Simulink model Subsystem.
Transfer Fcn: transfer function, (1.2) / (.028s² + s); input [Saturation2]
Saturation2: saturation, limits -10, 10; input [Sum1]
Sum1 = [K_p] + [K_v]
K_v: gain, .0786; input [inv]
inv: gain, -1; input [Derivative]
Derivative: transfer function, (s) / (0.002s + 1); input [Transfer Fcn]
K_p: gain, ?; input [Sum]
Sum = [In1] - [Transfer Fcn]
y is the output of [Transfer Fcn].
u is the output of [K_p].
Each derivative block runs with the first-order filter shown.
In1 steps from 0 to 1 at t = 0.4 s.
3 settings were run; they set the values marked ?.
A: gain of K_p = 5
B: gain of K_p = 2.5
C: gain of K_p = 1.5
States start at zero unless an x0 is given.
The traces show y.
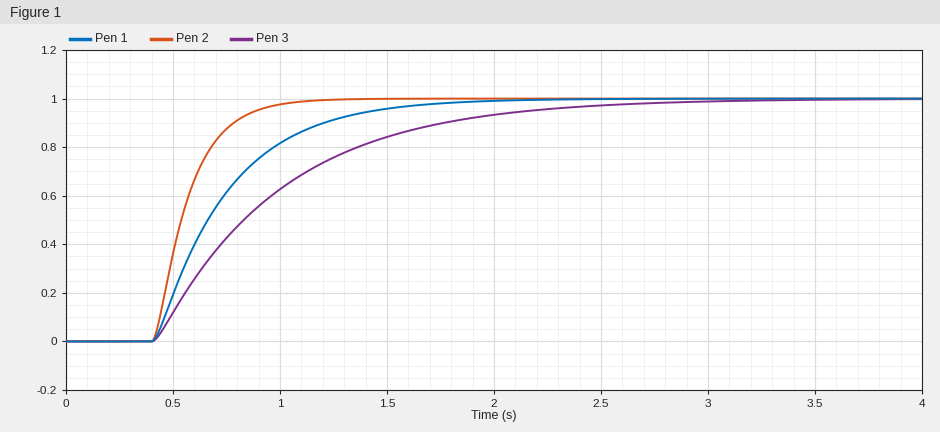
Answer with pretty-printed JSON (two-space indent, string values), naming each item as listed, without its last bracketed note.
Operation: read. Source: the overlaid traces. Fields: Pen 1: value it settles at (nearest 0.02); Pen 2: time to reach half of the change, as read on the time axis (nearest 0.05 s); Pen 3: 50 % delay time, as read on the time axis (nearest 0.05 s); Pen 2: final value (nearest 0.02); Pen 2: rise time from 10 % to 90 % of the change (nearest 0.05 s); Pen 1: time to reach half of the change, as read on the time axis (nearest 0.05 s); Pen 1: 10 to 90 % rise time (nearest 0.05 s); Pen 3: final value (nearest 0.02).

{
  "Pen 1: value it settles at": "1.00",
  "Pen 2: time to reach half of the change, as read on the time axis": "0.55 s",
  "Pen 3: 50 % delay time, as read on the time axis": "0.85 s",
  "Pen 2: final value": "1.00",
  "Pen 2: rise time from 10 % to 90 % of the change": "0.35 s",
  "Pen 1: time to reach half of the change, as read on the time axis": "0.65 s",
  "Pen 1: 10 to 90 % rise time": "0.75 s",
  "Pen 3: final value": "1.00"
}
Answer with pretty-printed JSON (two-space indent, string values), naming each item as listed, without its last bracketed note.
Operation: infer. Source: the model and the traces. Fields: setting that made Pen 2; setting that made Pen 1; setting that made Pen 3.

{
  "setting that made Pen 2": "A",
  "setting that made Pen 1": "B",
  "setting that made Pen 3": "C"
}
